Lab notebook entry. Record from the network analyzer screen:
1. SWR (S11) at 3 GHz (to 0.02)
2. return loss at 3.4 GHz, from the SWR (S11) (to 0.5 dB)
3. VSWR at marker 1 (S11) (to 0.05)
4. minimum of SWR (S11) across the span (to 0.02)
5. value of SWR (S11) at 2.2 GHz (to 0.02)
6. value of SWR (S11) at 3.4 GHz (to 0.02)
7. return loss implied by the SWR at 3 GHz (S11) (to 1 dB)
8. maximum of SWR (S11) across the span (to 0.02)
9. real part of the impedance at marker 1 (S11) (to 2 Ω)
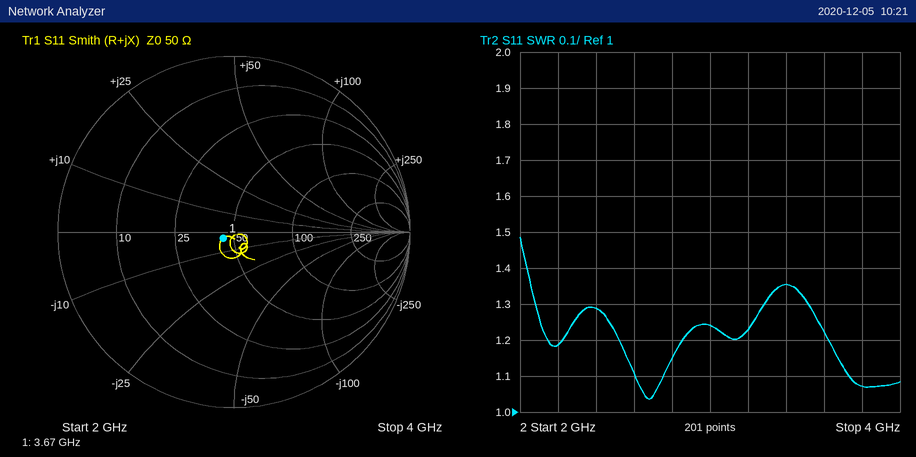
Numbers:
1.24
16.5 dB
1.15
1.04
1.18
1.36
19 dB
1.48
44 Ω
